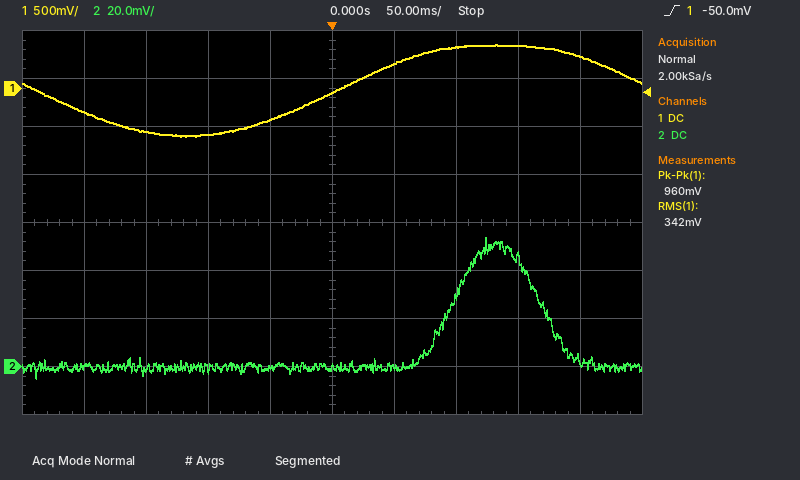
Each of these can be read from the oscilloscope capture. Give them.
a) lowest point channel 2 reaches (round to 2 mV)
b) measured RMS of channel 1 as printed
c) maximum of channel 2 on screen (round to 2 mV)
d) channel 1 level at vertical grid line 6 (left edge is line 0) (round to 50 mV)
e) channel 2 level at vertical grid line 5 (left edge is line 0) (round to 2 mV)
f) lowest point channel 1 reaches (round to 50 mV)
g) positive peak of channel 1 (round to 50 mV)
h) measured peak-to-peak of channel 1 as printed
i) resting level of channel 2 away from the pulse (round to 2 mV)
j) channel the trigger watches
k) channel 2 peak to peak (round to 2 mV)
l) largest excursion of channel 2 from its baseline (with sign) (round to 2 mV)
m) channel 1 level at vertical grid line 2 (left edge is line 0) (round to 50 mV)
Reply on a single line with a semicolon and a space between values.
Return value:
-4 mV; 342 mV; 54 mV; 250 mV; 0 mV; -500 mV; 450 mV; 960 mV; 0 mV; channel 1; 58 mV; +54 mV; -450 mV
